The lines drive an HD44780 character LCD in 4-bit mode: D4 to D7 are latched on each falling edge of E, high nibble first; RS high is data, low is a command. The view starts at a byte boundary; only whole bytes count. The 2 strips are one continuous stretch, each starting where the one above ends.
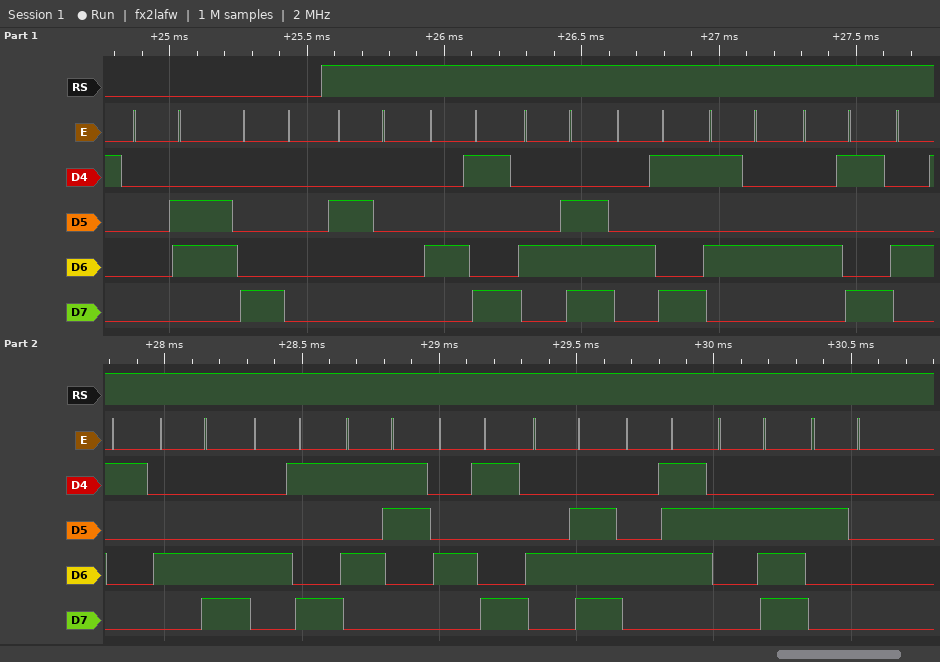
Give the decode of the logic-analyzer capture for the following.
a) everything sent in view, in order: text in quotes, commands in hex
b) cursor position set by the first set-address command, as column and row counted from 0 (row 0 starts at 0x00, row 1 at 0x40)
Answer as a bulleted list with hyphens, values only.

- 0x06 0x80 " INITIALISING. "
- column 0, row 0
